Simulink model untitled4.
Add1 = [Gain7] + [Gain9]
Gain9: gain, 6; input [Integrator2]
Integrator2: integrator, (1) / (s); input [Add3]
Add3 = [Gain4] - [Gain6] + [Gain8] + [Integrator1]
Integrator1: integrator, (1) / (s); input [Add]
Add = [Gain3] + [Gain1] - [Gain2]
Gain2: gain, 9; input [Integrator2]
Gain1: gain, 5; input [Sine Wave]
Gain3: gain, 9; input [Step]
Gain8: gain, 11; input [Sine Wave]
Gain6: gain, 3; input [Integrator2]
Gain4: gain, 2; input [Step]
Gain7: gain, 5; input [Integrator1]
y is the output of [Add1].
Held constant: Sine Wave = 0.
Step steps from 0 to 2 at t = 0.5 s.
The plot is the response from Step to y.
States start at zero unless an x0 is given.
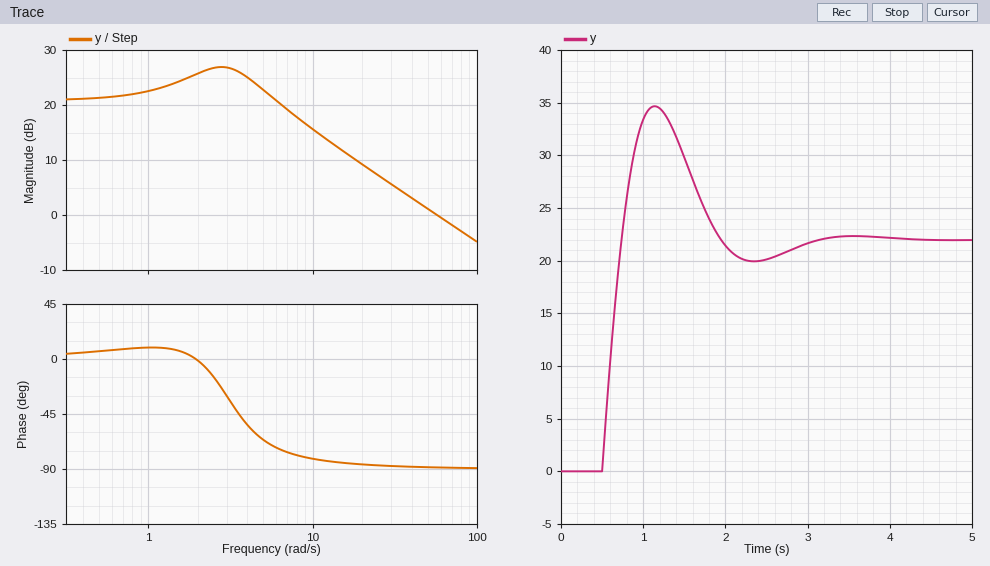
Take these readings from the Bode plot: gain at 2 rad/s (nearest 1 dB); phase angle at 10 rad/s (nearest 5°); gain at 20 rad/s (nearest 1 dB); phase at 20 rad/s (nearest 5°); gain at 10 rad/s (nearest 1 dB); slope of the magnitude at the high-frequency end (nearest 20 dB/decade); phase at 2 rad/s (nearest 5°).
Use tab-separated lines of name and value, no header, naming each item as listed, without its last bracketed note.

gain at 2 rad/s	26 dB
phase angle at 10 rad/s	-80°
gain at 20 rad/s	9 dB
phase at 20 rad/s	-85°
gain at 10 rad/s	16 dB
slope of the magnitude at the high-frequency end	-20 dB/decade
phase at 2 rad/s	0°
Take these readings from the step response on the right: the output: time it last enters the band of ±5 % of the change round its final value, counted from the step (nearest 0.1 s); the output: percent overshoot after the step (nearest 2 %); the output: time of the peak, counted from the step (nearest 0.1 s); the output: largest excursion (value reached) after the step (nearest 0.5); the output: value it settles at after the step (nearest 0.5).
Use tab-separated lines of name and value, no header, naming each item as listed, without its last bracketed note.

the output: time it last enters the band of ±5 % of the change round its final value, counted from the step	2.3 s
the output: percent overshoot after the step	58 %
the output: time of the peak, counted from the step	0.6 s
the output: largest excursion (value reached) after the step	34.5
the output: value it settles at after the step	22.0
